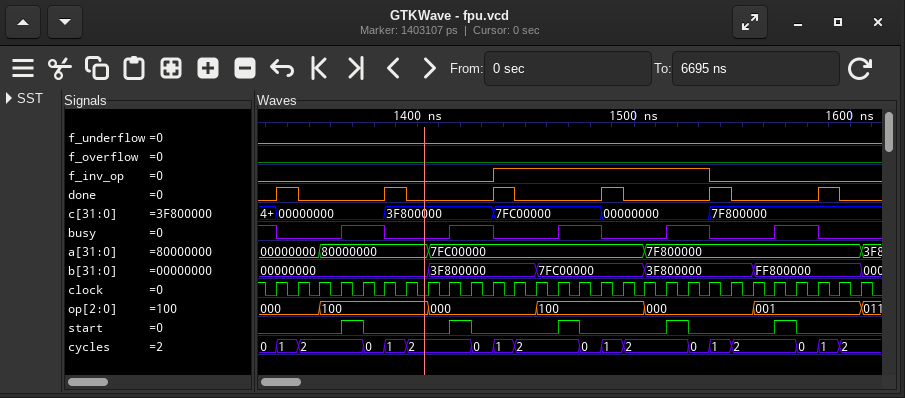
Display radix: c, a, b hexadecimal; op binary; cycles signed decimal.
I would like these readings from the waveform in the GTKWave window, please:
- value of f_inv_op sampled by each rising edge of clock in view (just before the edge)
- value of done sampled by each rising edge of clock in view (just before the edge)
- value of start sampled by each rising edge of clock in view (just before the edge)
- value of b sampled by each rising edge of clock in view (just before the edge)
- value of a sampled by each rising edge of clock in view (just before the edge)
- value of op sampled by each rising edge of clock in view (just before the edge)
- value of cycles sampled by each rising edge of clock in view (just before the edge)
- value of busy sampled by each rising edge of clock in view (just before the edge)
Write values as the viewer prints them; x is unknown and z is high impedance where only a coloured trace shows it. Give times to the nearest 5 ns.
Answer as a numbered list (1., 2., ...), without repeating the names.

1. 0 0 0 0 0 0 0 0 0 0 0 1 1 1 1 1 1 1 1 1 1 0 0 0 0 0 0 0
2. 0 1 0 0 0 0 1 0 0 0 0 1 0 0 0 0 1 0 0 0 0 1 0 0 0 0 1 0
3. 0 0 0 0 1 0 0 0 0 1 0 0 0 0 1 0 0 0 0 1 0 0 0 0 1 0 0 0
4. 00000000, 00000000, 00000000, 00000000, 00000000, 00000000, 00000000, 00000000, 3F800000, 3F800000, 3F800000, 3F800000, 3F800000, 7FC00000, 7FC00000, 7FC00000, 7FC00000, 7FC00000, 3F800000, 3F800000, 3F800000, 3F800000, 3F800000, FF800000, FF800000, FF800000, FF800000, FF800000
5. 00000000, 00000000, 00000000, 80000000, 80000000, 80000000, 80000000, 80000000, 7FC00000, 7FC00000, 7FC00000, 7FC00000, 7FC00000, 7FC00000, 7FC00000, 7FC00000, 7FC00000, 7FC00000, 7F800000, 7F800000, 7F800000, 7F800000, 7F800000, 7F800000, 7F800000, 7F800000, 7F800000, 7F800000
6. 000, 000, 000, 100, 100, 100, 100, 100, 000, 000, 000, 000, 000, 100, 100, 100, 100, 100, 000, 000, 000, 000, 000, 001, 001, 001, 001, 001
7. 0, 1, 2, 2, 2, 0, 1, 2, 2, 2, 0, 1, 2, 2, 2, 0, 1, 2, 2, 2, 0, 1, 2, 2, 2, 0, 1, 2
8. 1 0 0 0 1 1 0 0 0 1 1 0 0 0 1 1 0 0 0 1 1 0 0 0 1 1 0 0
